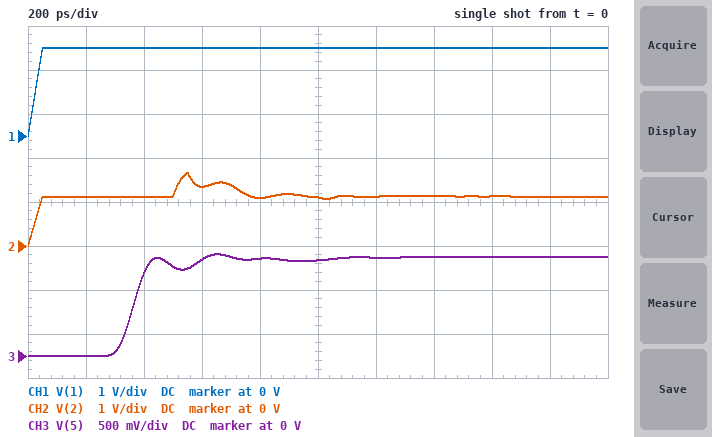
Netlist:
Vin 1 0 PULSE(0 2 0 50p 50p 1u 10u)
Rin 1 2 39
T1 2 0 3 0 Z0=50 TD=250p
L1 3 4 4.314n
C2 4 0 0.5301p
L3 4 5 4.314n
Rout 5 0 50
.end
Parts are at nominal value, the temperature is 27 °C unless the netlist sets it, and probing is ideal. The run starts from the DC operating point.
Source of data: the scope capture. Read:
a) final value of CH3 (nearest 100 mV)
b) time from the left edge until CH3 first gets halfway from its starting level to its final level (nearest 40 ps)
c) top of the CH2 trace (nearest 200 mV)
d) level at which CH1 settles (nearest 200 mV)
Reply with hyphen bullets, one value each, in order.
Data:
- 1.1 V
- 360 ps
- 1.6 V
- 2.0 V
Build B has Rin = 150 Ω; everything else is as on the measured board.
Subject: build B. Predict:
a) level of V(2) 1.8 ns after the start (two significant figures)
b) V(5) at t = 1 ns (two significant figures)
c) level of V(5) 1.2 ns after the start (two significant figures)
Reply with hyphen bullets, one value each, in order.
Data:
- 500 mV
- 550 mV
- 510 mV
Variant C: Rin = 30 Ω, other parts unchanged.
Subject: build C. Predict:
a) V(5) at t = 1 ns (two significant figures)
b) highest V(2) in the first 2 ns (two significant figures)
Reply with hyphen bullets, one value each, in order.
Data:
- 1.2 V
- 1.8 V
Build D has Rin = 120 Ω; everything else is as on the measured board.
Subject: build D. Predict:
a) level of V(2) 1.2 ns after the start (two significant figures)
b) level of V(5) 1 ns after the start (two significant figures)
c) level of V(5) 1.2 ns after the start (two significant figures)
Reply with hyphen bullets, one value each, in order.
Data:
- 580 mV
- 640 mV
- 600 mV
